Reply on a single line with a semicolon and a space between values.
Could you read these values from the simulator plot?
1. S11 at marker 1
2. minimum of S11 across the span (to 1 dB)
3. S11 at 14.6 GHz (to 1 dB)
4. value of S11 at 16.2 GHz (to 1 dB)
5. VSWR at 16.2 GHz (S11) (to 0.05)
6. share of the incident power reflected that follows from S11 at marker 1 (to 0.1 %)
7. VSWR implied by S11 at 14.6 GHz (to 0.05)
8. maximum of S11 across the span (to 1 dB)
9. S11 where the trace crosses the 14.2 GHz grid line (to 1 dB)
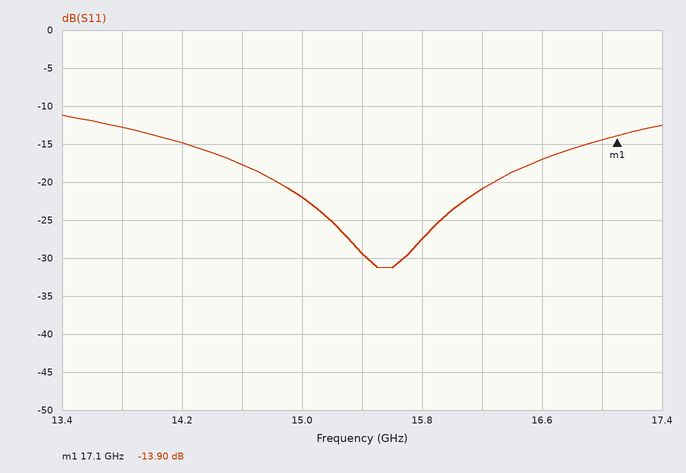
-13.90 dB; -31 dB; -18 dB; -21 dB; 1.20; 4.1 %; 1.30; -11 dB; -15 dB
